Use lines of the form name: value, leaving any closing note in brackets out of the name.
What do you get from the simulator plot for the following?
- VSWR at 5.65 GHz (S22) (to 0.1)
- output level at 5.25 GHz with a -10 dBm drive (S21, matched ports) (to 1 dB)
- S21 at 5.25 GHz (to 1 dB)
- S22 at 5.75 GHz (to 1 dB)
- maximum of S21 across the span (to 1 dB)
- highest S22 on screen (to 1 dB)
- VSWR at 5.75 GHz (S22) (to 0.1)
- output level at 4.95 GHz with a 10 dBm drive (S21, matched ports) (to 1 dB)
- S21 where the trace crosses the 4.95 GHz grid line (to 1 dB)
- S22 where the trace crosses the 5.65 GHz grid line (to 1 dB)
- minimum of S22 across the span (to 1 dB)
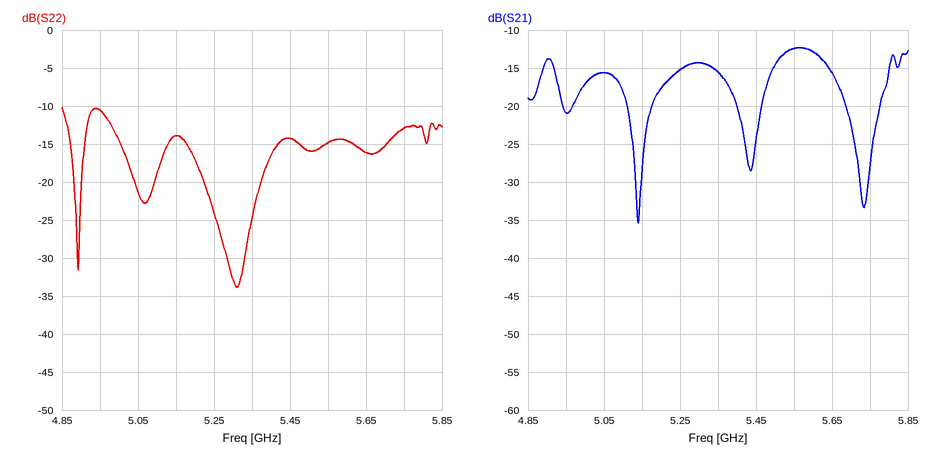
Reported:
VSWR at 5.65 GHz (S22): 1.4
output level at 5.25 GHz with a -10 dBm drive (S21, matched ports): -25 dBm
S21 at 5.25 GHz: -15 dB
S22 at 5.75 GHz: -13 dB
maximum of S21 across the span: -12 dB
highest S22 on screen: -10 dB
VSWR at 5.75 GHz (S22): 1.6
output level at 4.95 GHz with a 10 dBm drive (S21, matched ports): -11 dBm
S21 where the trace crosses the 4.95 GHz grid line: -21 dB
S22 where the trace crosses the 5.65 GHz grid line: -16 dB
minimum of S22 across the span: -34 dB
